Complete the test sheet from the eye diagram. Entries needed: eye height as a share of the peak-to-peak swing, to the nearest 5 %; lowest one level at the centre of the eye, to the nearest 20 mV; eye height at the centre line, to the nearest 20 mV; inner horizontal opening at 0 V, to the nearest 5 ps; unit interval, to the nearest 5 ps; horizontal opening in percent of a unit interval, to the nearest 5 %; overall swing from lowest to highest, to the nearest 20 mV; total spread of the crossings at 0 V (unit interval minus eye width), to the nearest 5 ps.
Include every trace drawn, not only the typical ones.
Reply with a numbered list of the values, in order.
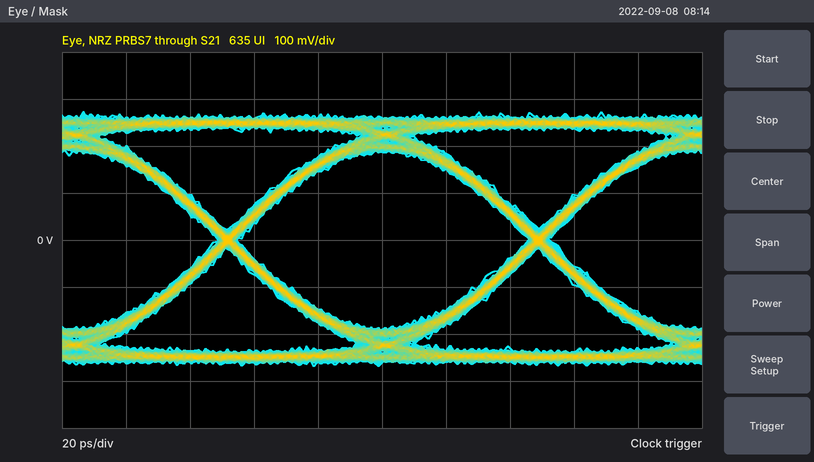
1. 70 %
2. 180 mV
3. 380 mV
4. 90 ps
5. 95 ps
6. 95 %
7. 540 mV
8. 5 ps
